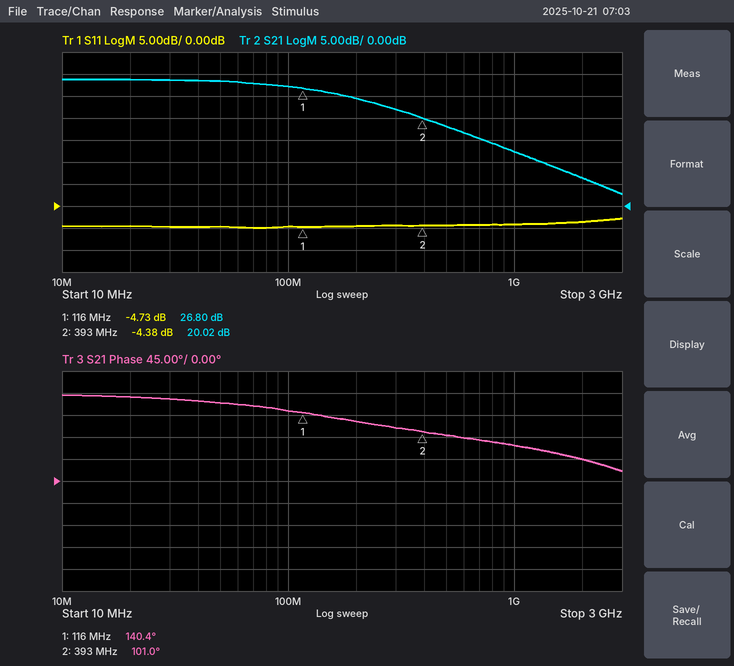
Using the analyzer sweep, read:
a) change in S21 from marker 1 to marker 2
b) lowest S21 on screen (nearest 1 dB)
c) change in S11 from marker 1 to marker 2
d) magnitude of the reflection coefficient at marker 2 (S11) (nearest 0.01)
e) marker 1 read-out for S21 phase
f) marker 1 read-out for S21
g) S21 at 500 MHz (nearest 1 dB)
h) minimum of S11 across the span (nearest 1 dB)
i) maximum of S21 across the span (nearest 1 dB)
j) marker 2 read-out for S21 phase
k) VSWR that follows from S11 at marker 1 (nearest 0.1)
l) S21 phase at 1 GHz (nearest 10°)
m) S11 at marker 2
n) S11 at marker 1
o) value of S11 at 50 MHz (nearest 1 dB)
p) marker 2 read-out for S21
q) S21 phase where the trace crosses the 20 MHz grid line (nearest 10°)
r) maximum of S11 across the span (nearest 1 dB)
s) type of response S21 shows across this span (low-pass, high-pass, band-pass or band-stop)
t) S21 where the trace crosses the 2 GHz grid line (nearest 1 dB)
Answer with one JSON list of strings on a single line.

["-6.78 dB", "3 dB", "0.35 dB", "0.60", "140.4°", "26.80 dB", "18 dB", "-5 dB", "29 dB", "101.0°", "3.8", "70°", "-4.38 dB", "-4.73 dB", "-5 dB", "20.02 dB", "170°", "-3 dB", "low-pass", "6 dB"]
